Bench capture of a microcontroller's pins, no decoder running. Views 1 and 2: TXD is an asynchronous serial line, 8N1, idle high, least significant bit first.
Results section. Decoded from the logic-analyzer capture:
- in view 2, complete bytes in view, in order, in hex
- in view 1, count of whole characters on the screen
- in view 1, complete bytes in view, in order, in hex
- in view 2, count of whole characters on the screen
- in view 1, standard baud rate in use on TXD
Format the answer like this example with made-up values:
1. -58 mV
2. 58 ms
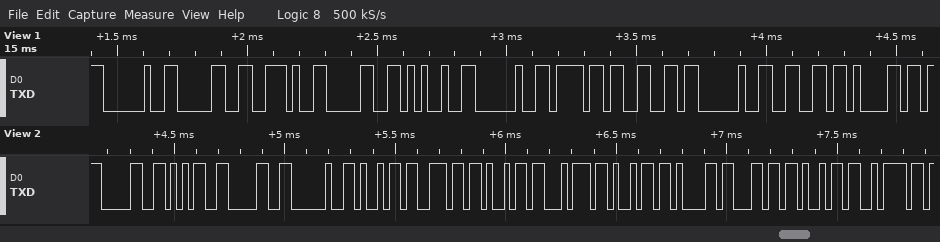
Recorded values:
1. 30 35 30 20 69 6E 69 74 69 61 6C 69 7A
2. 11
3. 20 30 2E 30 25 20 6F 66 20 66 61
4. 13
5. 38400 baud
